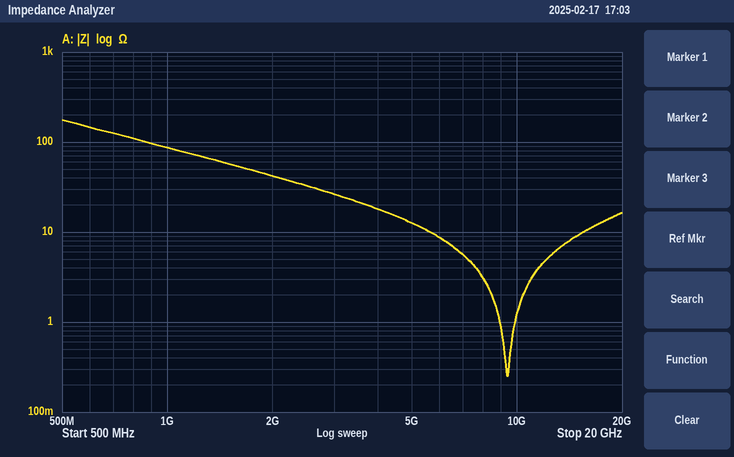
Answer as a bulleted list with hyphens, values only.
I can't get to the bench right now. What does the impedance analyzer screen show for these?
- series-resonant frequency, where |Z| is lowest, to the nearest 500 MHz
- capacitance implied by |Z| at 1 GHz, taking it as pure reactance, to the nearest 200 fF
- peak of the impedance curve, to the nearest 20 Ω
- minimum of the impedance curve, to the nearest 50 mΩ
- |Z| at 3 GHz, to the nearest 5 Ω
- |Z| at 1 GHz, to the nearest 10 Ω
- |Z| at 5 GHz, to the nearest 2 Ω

- 9.5 GHz
- 1.8 pF
- 180 Ω
- 250 mΩ
- 25 Ω
- 90 Ω
- 12 Ω
